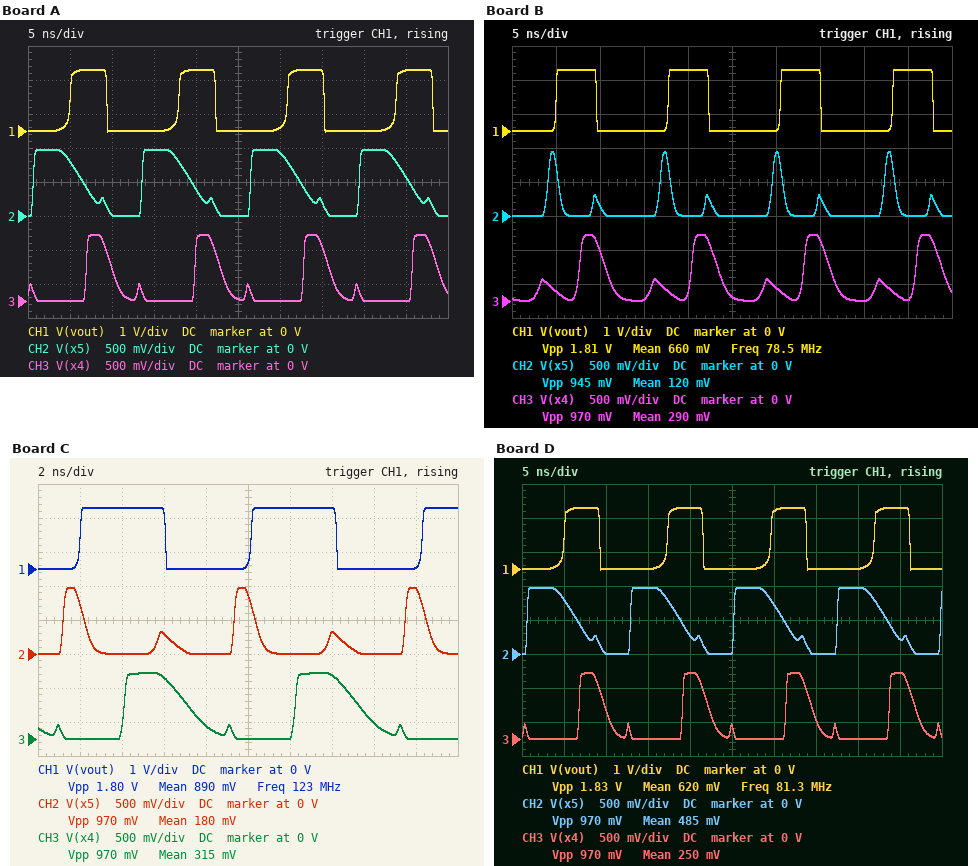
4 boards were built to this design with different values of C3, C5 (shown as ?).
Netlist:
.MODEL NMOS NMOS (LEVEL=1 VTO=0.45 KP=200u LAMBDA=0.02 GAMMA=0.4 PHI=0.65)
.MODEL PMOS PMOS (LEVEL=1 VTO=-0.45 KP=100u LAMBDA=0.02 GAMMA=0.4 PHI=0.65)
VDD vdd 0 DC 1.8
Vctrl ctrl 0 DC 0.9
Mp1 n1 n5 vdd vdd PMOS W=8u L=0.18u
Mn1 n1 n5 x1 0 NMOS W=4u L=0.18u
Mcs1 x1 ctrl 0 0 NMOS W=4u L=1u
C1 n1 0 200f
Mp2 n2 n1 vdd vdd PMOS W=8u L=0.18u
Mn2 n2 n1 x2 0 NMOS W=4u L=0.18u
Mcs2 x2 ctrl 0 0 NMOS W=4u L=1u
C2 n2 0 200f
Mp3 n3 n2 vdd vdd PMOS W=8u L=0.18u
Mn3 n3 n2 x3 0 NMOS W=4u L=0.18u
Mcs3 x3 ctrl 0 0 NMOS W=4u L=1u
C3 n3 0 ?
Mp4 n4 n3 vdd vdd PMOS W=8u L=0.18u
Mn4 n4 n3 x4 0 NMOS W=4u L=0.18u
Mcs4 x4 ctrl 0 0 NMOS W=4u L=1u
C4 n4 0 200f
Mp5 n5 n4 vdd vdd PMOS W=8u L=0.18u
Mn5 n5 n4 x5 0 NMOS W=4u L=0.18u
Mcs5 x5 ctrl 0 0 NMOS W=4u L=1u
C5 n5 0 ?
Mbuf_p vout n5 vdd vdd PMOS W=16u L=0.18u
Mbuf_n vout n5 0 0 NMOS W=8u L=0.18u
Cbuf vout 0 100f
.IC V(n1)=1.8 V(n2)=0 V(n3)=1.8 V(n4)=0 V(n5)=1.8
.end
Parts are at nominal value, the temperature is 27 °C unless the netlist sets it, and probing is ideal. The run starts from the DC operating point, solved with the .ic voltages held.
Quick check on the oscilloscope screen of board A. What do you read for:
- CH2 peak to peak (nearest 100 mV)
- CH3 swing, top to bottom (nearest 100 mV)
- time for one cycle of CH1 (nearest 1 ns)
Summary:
1.0 V
1.0 V
13 ns
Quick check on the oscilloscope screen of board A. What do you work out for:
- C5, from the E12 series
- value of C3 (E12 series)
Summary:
390 fF
150 fF
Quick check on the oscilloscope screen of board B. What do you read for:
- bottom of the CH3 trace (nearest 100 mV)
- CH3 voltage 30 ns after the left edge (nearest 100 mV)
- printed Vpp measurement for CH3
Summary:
0 V
200 mV
970 mV
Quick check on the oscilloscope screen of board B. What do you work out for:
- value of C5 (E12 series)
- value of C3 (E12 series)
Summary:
82 fF
470 fF
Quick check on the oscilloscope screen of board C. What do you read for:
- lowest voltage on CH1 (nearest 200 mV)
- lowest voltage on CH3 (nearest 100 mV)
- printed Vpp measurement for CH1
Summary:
0 V
0 V
1.80 V
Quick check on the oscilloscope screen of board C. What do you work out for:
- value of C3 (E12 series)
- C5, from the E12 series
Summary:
68 fF
68 fF
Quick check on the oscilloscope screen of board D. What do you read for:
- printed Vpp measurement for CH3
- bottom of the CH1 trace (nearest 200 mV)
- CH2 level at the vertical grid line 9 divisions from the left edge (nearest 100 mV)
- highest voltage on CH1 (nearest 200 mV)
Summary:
970 mV
0 V
200 mV
1.8 V
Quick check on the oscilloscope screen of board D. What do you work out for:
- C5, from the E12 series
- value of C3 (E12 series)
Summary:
390 fF
100 fF
